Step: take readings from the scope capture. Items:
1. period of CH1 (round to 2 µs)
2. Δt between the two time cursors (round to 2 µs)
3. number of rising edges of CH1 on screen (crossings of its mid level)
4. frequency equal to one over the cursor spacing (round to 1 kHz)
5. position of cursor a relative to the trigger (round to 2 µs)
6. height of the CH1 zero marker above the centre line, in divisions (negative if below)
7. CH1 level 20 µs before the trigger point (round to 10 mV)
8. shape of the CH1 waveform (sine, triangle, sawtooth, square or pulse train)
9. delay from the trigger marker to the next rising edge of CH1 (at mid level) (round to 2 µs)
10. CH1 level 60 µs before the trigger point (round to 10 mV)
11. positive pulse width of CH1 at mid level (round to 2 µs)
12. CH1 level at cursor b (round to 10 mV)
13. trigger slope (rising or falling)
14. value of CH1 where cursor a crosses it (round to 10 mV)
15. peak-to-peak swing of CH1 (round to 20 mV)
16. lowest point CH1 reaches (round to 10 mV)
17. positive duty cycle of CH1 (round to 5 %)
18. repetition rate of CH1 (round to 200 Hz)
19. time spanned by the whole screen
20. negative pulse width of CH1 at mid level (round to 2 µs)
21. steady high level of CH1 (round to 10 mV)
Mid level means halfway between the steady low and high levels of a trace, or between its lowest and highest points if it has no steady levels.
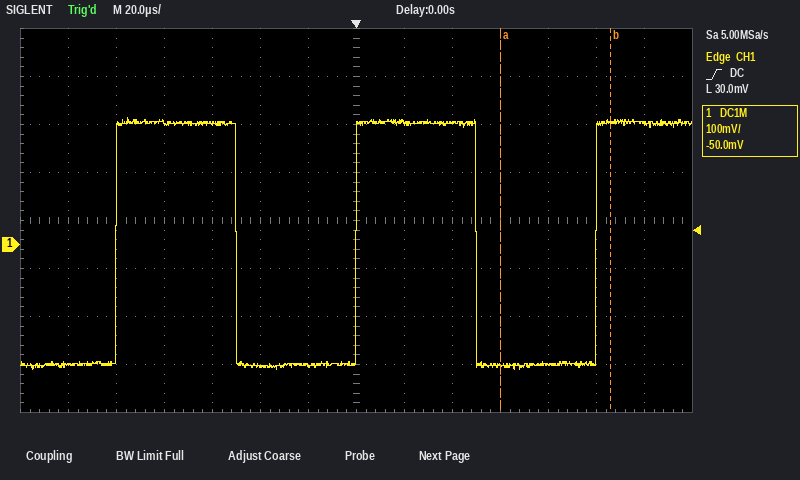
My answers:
100 µs
46 µs
3
22 kHz
+60 µs
-0.5 div
-250 mV
square
100 µs
250 mV
50 µs
260 mV
rising
-250 mV
520 mV
-260 mV
50 %
10.0 kHz
280 µs
50 µs
250 mV
